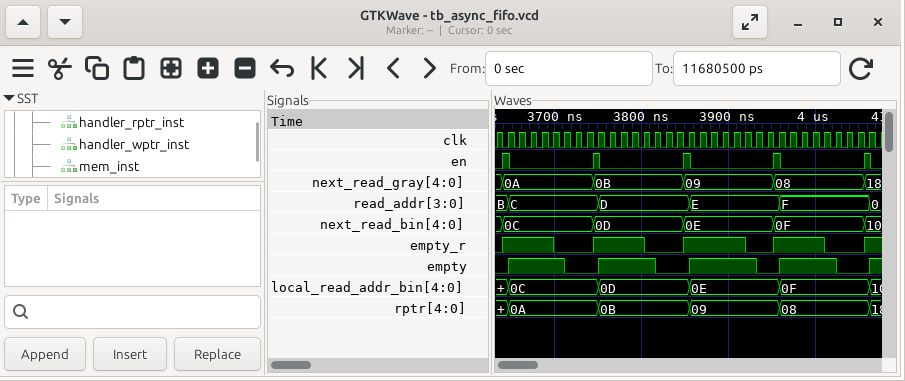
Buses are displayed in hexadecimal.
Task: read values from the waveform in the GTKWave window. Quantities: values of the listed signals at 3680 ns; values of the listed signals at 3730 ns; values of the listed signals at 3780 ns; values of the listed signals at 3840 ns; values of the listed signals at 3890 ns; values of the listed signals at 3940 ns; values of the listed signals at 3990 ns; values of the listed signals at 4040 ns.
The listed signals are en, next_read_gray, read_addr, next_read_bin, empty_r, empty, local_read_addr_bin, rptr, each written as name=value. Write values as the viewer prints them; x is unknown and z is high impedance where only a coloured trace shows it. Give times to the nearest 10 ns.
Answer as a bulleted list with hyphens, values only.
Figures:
- en=0, next_read_gray=0A, read_addr=C, next_read_bin=0C, empty_r=1, empty=1, local_read_addr_bin=0C, rptr=0A
- en=0, next_read_gray=0A, read_addr=C, next_read_bin=0C, empty_r=0, empty=0, local_read_addr_bin=0C, rptr=0A
- en=0, next_read_gray=0B, read_addr=D, next_read_bin=0D, empty_r=1, empty=1, local_read_addr_bin=0D, rptr=0B
- en=0, next_read_gray=0B, read_addr=D, next_read_bin=0D, empty_r=0, empty=0, local_read_addr_bin=0D, rptr=0B
- en=0, next_read_gray=09, read_addr=E, next_read_bin=0E, empty_r=1, empty=1, local_read_addr_bin=0E, rptr=09
- en=0, next_read_gray=09, read_addr=E, next_read_bin=0E, empty_r=0, empty=0, local_read_addr_bin=0E, rptr=09
- en=0, next_read_gray=08, read_addr=F, next_read_bin=0F, empty_r=1, empty=1, local_read_addr_bin=0F, rptr=08
- en=0, next_read_gray=08, read_addr=F, next_read_bin=0F, empty_r=0, empty=0, local_read_addr_bin=0F, rptr=08
